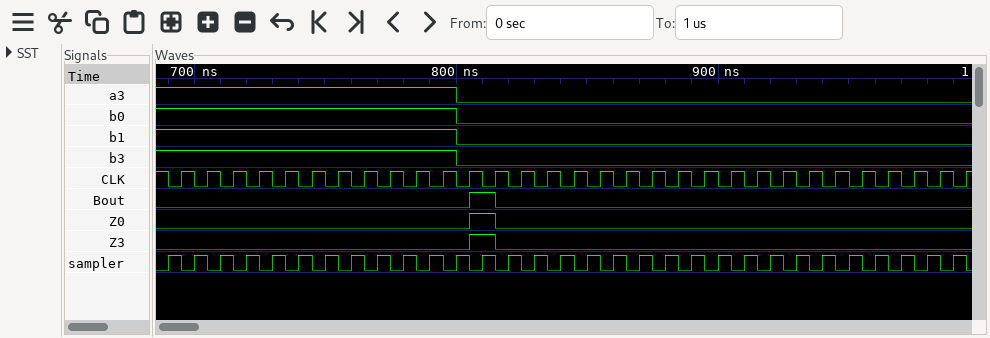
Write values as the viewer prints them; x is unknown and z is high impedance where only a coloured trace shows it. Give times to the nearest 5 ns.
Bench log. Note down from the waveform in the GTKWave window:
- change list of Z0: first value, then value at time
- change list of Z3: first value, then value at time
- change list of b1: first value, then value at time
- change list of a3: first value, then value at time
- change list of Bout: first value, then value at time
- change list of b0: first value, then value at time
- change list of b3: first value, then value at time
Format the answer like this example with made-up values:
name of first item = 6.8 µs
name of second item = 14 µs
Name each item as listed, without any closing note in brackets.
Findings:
change list of Z0: first value, then value at time = 0, 1 at 805 ns, 0 at 815 ns
change list of Z3: first value, then value at time = 0, 1 at 805 ns, 0 at 815 ns
change list of b1: first value, then value at time = 1, 0 at 800 ns
change list of a3: first value, then value at time = 1, 0 at 800 ns
change list of Bout: first value, then value at time = 0, 1 at 805 ns, 0 at 815 ns
change list of b0: first value, then value at time = 1, 0 at 800 ns
change list of b3: first value, then value at time = 1, 0 at 800 ns
